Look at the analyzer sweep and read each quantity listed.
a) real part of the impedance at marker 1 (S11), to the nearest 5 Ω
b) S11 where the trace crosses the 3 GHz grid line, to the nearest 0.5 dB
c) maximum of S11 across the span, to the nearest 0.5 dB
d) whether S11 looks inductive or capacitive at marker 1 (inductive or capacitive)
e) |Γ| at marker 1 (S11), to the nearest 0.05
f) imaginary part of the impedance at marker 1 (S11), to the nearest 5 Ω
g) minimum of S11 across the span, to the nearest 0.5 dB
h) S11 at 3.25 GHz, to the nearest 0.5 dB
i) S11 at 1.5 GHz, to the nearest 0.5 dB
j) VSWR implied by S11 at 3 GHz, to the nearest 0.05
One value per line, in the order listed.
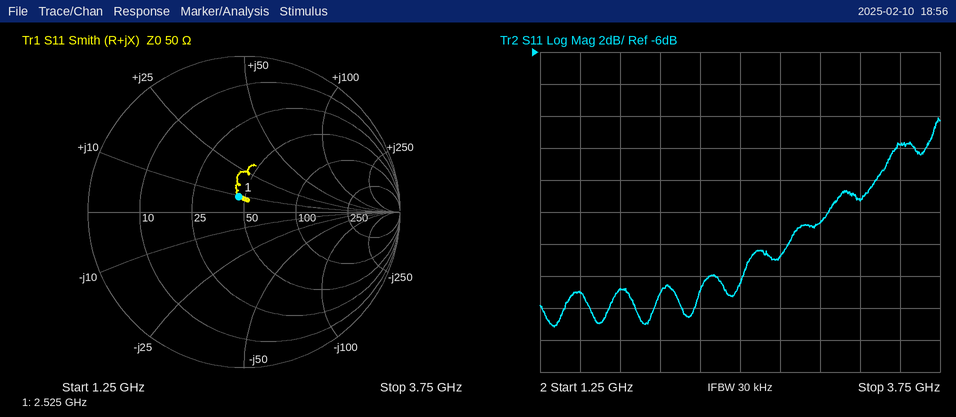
45 Ω
-16.5 dB
-10.0 dB
inductive
0.10
+10 Ω
-23.0 dB
-15.0 dB
-21.0 dB
1.35
